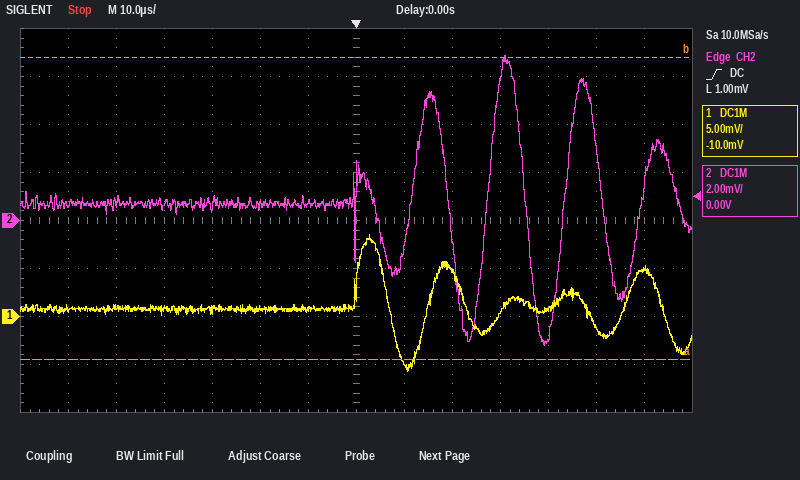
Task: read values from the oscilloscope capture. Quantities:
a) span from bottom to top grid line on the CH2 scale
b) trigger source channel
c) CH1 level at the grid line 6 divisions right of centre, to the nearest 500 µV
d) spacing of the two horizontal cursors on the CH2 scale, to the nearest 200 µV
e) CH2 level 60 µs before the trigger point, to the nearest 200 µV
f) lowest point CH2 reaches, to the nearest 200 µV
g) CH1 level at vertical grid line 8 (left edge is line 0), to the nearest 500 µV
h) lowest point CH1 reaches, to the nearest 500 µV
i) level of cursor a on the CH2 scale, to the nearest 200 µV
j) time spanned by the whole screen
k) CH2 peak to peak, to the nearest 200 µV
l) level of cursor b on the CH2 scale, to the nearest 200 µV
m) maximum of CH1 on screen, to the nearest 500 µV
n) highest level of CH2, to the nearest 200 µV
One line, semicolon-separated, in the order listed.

16 mV; CH2; 5.0 mV; 12.6 mV; 600 µV; -5.2 mV; -5.0 mV; -5.5 mV; -5.8 mV; 140 µs; 12.0 mV; 6.8 mV; 8.5 mV; 6.8 mV
